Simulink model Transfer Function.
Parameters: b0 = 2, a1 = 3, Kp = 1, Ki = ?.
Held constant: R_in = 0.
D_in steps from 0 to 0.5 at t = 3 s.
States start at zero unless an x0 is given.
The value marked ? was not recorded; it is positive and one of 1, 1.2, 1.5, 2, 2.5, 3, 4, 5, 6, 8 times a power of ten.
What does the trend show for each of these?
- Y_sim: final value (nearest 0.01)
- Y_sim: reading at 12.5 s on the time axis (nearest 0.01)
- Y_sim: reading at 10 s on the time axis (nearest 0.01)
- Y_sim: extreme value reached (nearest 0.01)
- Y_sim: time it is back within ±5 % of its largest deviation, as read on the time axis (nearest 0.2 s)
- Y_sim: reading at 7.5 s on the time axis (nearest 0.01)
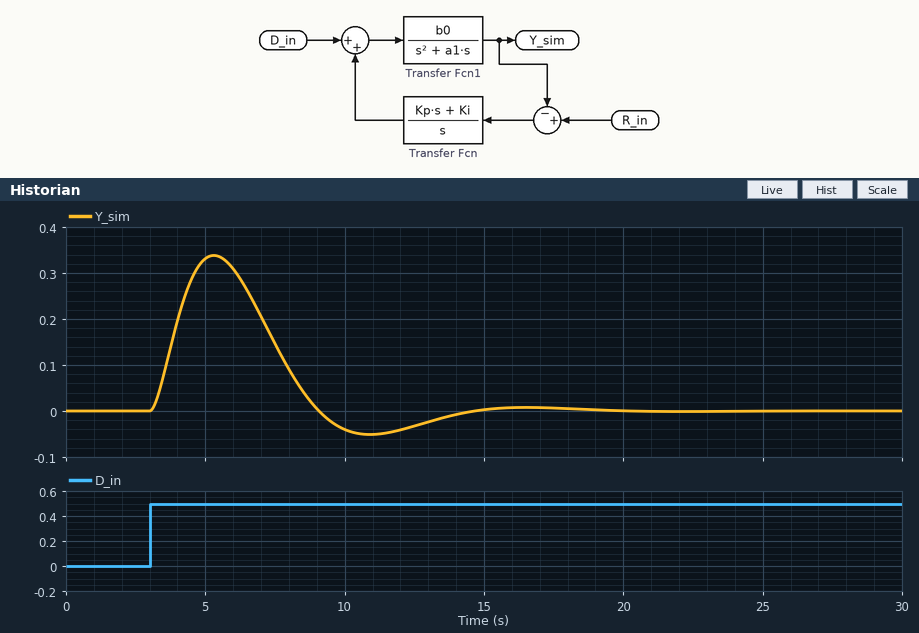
0.00
-0.03
-0.04
0.34
13.4 s
0.15
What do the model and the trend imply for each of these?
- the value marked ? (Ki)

0.5
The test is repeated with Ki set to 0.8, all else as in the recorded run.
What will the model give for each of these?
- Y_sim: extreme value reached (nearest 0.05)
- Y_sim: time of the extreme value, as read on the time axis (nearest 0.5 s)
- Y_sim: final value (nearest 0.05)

0.30
5.0 s
0.00
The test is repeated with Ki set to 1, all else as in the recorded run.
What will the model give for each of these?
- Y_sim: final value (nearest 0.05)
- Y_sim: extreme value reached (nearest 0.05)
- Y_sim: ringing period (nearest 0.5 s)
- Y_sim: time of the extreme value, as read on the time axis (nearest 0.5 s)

0.00
0.30
7.5 s
5.0 s
